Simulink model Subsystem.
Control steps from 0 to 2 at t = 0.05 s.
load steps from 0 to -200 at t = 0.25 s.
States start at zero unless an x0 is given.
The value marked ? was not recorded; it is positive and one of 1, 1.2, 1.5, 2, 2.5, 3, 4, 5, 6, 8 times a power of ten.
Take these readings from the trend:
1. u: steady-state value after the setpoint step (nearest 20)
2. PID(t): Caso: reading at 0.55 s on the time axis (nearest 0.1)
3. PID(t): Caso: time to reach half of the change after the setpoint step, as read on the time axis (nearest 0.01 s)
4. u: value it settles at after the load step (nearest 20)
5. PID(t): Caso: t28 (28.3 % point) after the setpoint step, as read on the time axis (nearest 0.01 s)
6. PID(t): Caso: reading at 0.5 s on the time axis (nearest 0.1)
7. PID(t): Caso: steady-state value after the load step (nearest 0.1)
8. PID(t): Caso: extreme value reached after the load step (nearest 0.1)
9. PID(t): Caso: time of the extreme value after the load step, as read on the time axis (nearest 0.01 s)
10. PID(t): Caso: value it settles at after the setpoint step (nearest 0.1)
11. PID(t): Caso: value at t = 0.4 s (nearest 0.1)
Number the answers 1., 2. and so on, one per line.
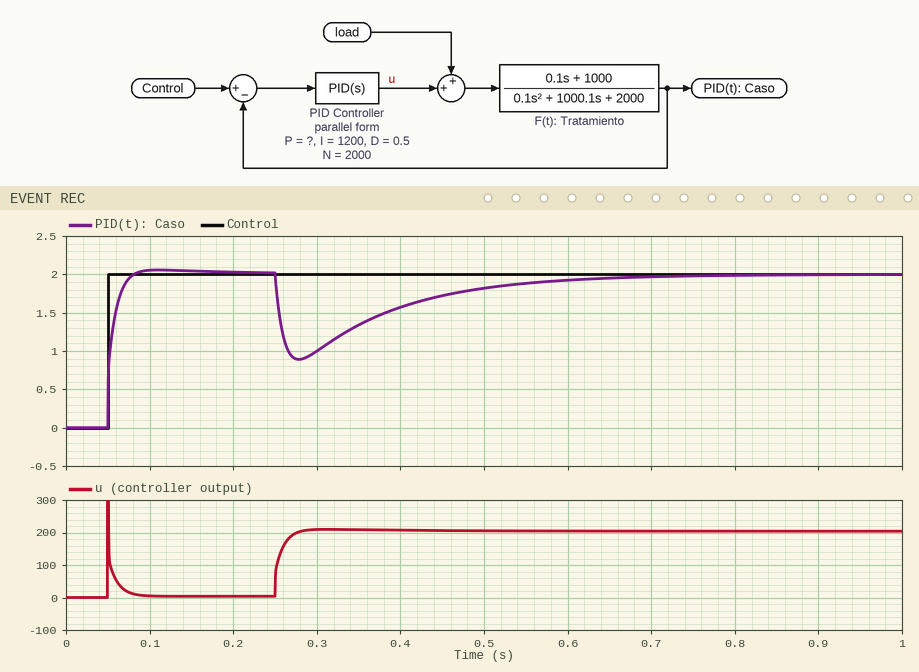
1. 0
2. 1.9
3. 0.05 s
4. 200
5. 0.05 s
6. 1.8
7. 2.0
8. 0.9
9. 0.28 s
10. 2.0
11. 1.6
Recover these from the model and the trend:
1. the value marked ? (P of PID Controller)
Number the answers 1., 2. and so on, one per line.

1. 150
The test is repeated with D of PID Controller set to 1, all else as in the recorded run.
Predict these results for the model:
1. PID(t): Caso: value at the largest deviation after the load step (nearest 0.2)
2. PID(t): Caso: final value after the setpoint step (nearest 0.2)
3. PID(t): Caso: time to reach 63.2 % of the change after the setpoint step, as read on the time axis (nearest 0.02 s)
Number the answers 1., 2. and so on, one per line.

1. 1.0
2. 2.0
3. 0.06 s
